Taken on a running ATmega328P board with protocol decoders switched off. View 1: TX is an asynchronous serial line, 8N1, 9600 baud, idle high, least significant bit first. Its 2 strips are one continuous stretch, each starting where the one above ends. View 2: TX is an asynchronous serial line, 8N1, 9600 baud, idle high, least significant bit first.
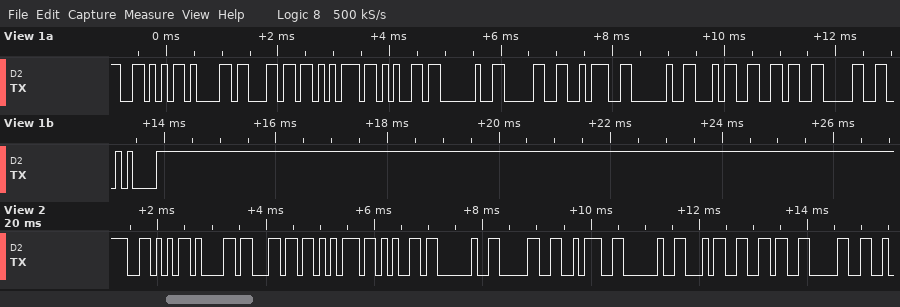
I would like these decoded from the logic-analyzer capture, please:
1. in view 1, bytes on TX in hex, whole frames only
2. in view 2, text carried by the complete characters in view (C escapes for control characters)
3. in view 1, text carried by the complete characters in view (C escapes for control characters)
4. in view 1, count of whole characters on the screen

56 61 6C 75 65 20 30 3A 20 34 36 30 0A
"Value 0: 460"
"Value 0: 460\n"
13
